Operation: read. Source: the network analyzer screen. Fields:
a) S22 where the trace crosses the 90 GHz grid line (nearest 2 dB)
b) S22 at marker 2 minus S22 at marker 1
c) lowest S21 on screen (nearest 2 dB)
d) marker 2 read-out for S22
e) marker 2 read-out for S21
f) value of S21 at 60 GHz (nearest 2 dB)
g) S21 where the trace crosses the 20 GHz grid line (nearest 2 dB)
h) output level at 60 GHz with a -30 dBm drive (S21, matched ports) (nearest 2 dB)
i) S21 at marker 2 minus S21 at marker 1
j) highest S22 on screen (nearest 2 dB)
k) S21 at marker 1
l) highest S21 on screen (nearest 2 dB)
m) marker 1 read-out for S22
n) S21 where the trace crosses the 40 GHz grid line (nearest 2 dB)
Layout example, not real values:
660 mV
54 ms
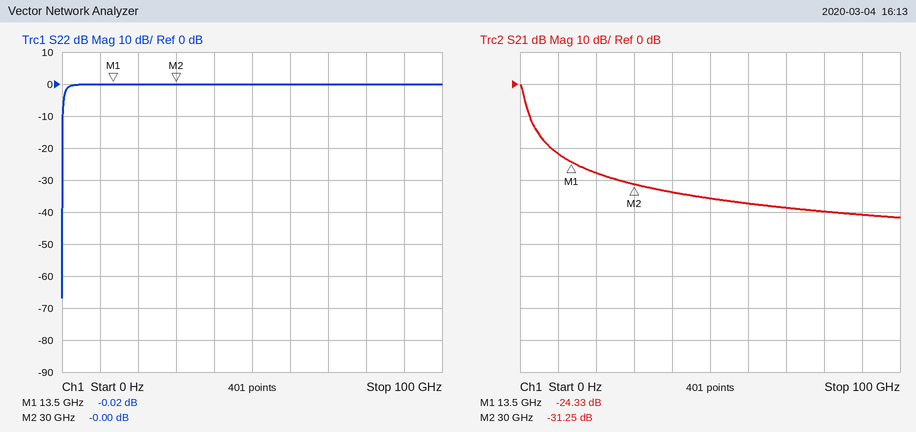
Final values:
0 dB
0.02 dB
-42 dB
-0.00 dB
-31.25 dB
-38 dB
-28 dB
-68 dBm
-6.92 dB
0 dB
-24.33 dB
0 dB
-0.02 dB
-34 dB
